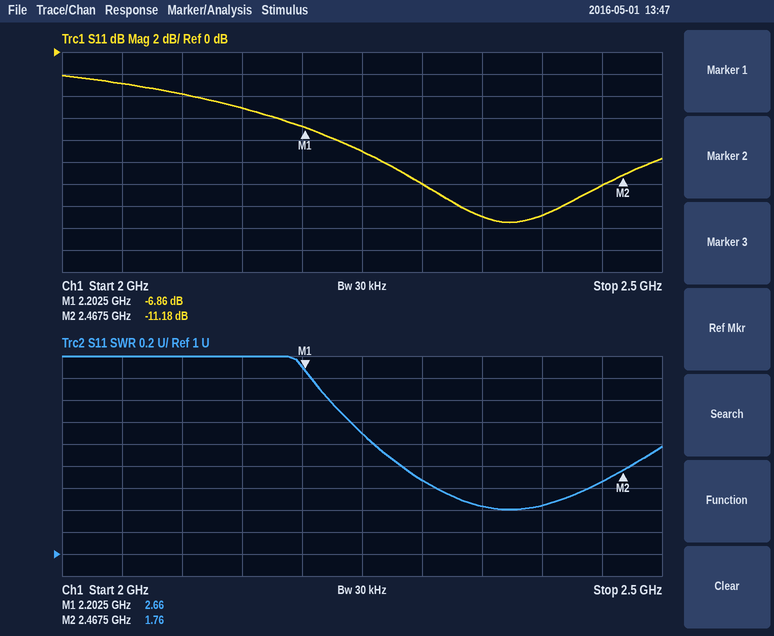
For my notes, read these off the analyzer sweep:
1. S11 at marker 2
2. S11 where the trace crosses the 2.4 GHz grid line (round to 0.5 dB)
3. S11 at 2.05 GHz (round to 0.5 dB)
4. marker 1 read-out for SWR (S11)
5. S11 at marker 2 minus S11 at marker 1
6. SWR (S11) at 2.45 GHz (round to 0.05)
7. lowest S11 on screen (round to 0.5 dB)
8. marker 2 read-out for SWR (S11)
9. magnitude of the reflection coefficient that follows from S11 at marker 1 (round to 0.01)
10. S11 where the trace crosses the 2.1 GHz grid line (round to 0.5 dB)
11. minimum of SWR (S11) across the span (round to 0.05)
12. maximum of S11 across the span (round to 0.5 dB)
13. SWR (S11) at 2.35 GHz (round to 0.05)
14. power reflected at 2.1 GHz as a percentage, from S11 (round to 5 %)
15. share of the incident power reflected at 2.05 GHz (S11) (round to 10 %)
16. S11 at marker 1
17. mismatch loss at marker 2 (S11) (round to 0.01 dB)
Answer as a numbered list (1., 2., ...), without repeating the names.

1. -11.18 dB
2. -15.0 dB
3. -3.0 dB
4. 2.66
5. -4.32 dB
6. 1.65
7. -15.5 dB
8. 1.76
9. 0.45
10. -4.0 dB
11. 1.40
12. -2.0 dB
13. 1.45
14. 40 %
15. 50 %
16. -6.86 dB
17. 0.34 dB
